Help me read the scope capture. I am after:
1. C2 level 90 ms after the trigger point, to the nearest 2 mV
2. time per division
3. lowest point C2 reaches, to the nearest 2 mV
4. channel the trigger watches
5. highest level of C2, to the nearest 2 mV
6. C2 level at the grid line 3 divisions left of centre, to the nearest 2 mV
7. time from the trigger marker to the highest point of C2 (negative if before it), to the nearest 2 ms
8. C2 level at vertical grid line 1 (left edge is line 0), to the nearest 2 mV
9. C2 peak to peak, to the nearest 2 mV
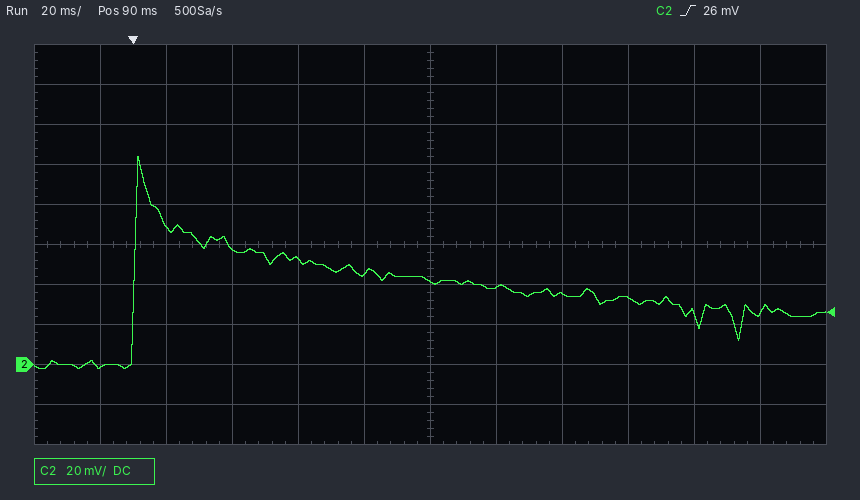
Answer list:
42 mV
20 ms
-2 mV
C2
104 mV
58 mV
+2 ms
-2 mV
106 mV
